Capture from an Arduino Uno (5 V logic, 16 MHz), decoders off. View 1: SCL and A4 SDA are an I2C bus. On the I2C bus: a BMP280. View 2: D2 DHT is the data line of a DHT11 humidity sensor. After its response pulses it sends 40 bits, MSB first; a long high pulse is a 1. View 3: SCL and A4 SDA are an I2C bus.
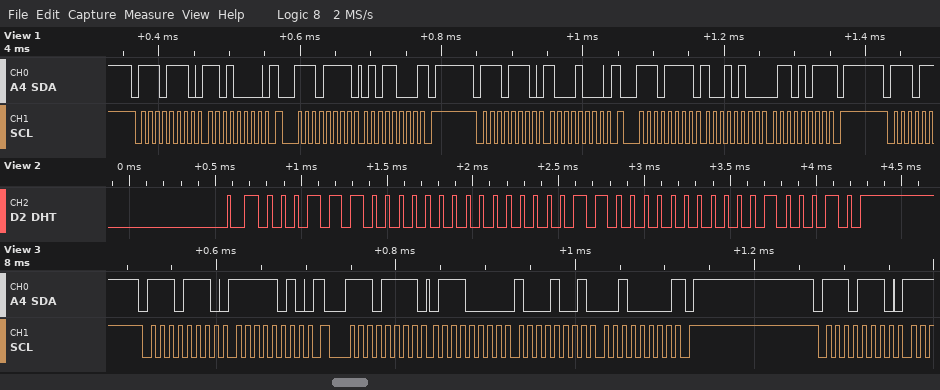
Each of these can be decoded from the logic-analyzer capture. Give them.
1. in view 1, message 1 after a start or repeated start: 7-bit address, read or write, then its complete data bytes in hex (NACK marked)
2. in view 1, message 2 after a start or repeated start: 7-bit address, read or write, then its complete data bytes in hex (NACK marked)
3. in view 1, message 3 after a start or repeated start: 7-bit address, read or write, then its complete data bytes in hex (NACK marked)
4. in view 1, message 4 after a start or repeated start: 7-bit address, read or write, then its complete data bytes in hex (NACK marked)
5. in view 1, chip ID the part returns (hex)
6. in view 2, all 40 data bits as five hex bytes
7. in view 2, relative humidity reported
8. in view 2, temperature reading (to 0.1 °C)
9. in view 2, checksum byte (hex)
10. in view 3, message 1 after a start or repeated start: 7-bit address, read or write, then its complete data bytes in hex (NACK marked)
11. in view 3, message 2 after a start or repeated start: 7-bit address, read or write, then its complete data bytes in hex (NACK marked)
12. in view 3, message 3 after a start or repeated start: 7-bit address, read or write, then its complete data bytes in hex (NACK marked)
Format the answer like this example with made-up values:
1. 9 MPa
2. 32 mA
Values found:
1. 0x77 write: D0
2. 0x77 read: 58 NACK
3. 0x77 write: 88
4. 0x77 read: 94 6B NACK
5. 0x58
6. 1C 00 06 00 22
7. 28 %
8. 6.0 °C
9. 0x22
10. 0x77 write: FA
11. 0x77 read: 70 89 20 NACK
12. 0x77 write
